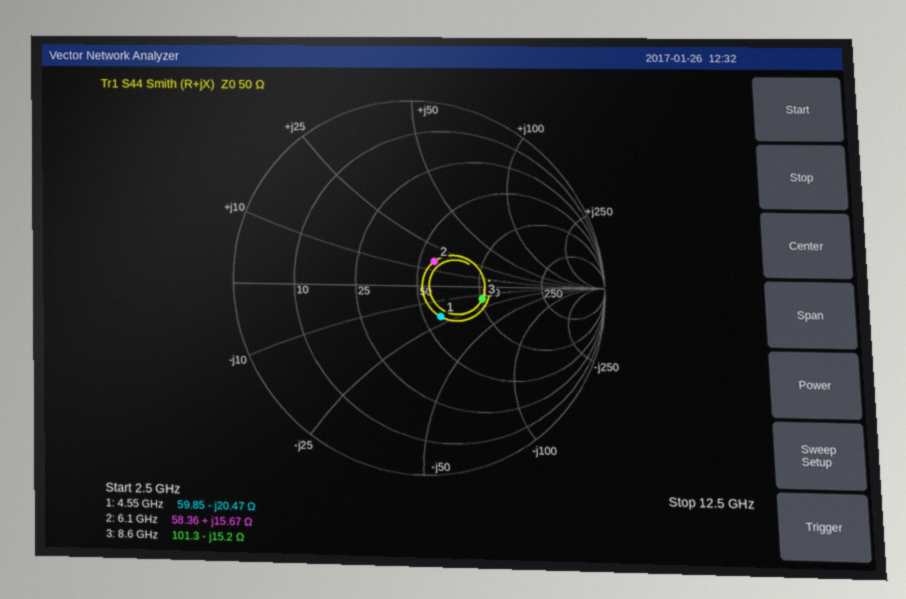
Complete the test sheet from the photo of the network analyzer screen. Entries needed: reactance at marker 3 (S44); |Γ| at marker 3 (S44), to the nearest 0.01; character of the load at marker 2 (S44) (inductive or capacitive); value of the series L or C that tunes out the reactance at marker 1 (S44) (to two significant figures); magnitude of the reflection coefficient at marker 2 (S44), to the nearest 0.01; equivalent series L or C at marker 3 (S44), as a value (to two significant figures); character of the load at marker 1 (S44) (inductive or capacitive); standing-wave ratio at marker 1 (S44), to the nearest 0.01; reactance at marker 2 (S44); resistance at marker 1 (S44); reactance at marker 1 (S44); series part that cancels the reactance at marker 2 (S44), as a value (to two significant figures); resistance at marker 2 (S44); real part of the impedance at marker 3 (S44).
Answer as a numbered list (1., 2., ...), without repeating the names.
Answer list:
1. -15.2 Ω
2. 0.35
3. inductive
4. 720 pH
5. 0.16
6. 1.2 pF
7. capacitive
8. 1.51
9. +15.67 Ω
10. 59.85 Ω
11. -20.47 Ω
12. 1.7 pF
13. 58.36 Ω
14. 101.3 Ω
